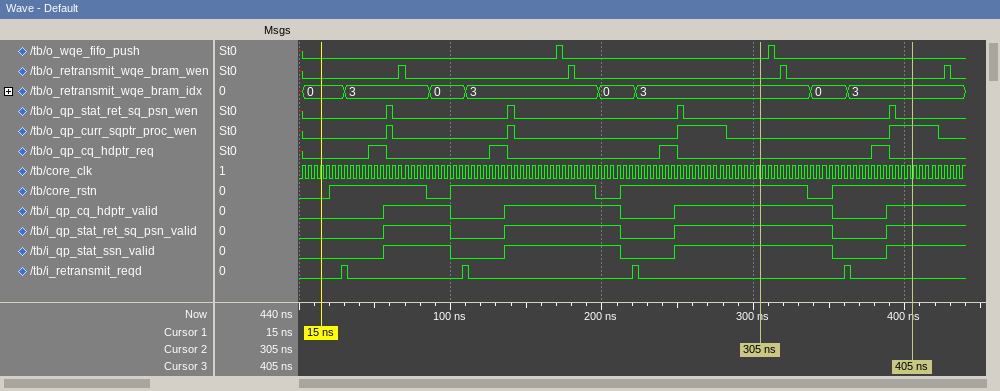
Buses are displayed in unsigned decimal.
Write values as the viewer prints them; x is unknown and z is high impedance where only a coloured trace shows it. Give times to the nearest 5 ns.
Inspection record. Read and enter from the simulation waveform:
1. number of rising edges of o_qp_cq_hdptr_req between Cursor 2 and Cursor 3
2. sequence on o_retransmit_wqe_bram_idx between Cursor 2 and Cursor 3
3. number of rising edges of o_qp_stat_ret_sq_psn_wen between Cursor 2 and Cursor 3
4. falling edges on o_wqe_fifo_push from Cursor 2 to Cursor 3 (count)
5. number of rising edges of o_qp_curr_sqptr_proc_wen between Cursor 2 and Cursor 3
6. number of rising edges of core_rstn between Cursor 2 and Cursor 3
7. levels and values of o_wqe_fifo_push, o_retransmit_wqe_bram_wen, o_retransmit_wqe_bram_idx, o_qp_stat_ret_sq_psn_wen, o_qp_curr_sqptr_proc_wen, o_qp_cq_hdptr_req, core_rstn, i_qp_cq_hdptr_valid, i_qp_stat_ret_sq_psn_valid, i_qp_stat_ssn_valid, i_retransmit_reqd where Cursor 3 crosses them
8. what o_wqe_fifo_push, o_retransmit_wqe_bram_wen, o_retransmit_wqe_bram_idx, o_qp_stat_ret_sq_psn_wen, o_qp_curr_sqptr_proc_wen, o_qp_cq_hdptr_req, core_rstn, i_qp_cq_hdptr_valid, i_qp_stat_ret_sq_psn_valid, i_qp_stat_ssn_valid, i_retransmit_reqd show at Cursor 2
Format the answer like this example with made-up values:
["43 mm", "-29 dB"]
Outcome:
["1", "3, 0, 3", "1", "1", "1", "1", "o_wqe_fifo_push=0, o_retransmit_wqe_bram_wen=0, o_retransmit_wqe_bram_idx=3, o_qp_stat_ret_sq_psn_wen=0, o_qp_curr_sqptr_proc_wen=1, o_qp_cq_hdptr_req=0, core_rstn=1, i_qp_cq_hdptr_valid=1, i_qp_stat_ret_sq_psn_valid=1, i_qp_stat_ssn_valid=1, i_retransmit_reqd=0", "o_wqe_fifo_push=0, o_retransmit_wqe_bram_wen=0, o_retransmit_wqe_bram_idx=3, o_qp_stat_ret_sq_psn_wen=0, o_qp_curr_sqptr_proc_wen=0, o_qp_cq_hdptr_req=0, core_rstn=1, i_qp_cq_hdptr_valid=1, i_qp_stat_ret_sq_psn_valid=1, i_qp_stat_ssn_valid=1, i_retransmit_reqd=0"]
